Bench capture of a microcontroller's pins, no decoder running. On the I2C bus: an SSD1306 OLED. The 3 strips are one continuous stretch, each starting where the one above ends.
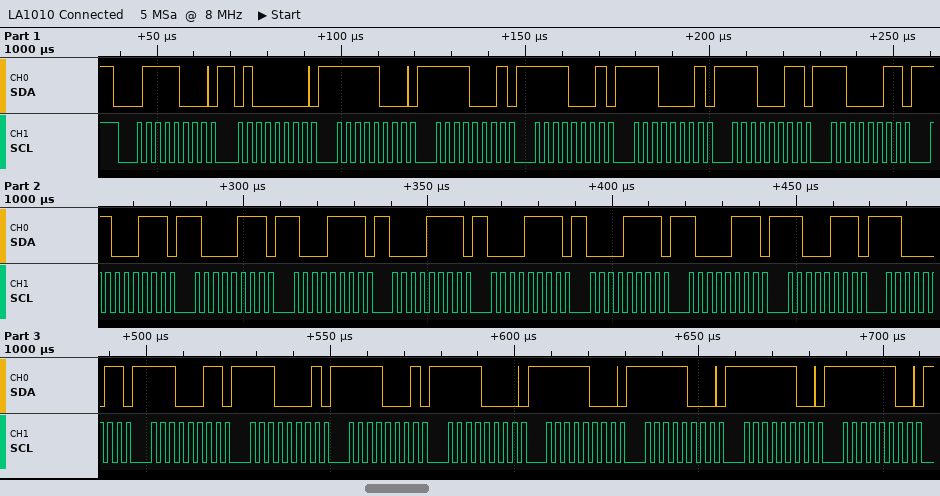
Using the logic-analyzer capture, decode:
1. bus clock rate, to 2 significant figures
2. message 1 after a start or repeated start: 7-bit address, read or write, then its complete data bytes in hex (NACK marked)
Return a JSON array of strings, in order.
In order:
["400 kHz", "0x3C write: 40 F8 F1 F1 E1 E3 C3 C7 87 8F 0F 0F 0F 87 C7 C3 E3 E1 F1 F0 F8 F8 FC FC"]
